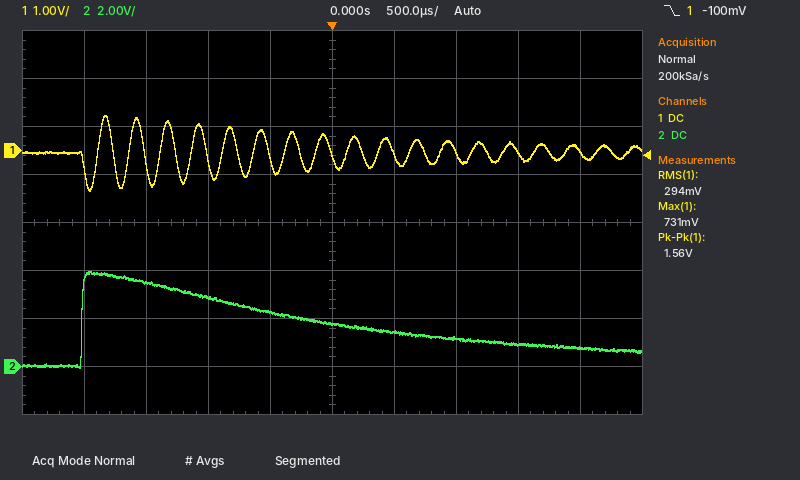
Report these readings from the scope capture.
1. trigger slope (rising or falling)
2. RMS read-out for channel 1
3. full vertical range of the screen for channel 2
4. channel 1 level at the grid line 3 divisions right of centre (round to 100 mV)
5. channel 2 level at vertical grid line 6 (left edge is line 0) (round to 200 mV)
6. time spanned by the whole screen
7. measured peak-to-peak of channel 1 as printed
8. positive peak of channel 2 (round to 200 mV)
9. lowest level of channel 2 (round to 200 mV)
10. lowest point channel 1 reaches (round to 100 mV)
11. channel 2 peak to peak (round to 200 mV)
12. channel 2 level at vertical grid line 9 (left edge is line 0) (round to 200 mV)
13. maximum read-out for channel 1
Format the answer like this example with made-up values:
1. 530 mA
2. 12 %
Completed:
1. falling
2. 294 mV
3. 16 V
4. 0.0 V
5. 1.4 V
6. 5 ms
7. 1.56 V
8. 4.0 V
9. 0.0 V
10. -800 mV
11. 4.0 V
12. 800 mV
13. 731 mV
